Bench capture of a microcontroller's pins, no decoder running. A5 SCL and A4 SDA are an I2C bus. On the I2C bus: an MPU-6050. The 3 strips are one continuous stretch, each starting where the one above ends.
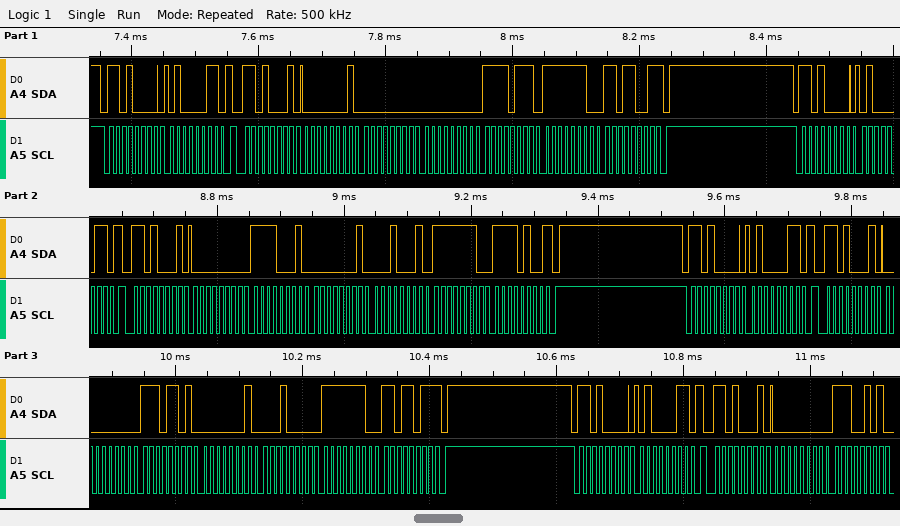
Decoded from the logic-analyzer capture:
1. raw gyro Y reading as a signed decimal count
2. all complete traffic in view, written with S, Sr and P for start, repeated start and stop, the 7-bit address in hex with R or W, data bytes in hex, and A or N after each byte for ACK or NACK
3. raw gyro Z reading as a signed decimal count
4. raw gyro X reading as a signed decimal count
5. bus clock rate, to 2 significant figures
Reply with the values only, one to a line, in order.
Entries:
247
S 68W A 43 A Sr 68R A 01 A 00 A 00 A F7 A FE A D9 N P S 68W A 43 A Sr 68R A 00 A F1 A 01 A 11 A FE A F4 N P S 68W A 43 A Sr 68R A 00 A ED A 01 A 10 A FE A DB N P S 68W A 43 A Sr 68R A 00 A E5 A
-295
256
100 kHz
